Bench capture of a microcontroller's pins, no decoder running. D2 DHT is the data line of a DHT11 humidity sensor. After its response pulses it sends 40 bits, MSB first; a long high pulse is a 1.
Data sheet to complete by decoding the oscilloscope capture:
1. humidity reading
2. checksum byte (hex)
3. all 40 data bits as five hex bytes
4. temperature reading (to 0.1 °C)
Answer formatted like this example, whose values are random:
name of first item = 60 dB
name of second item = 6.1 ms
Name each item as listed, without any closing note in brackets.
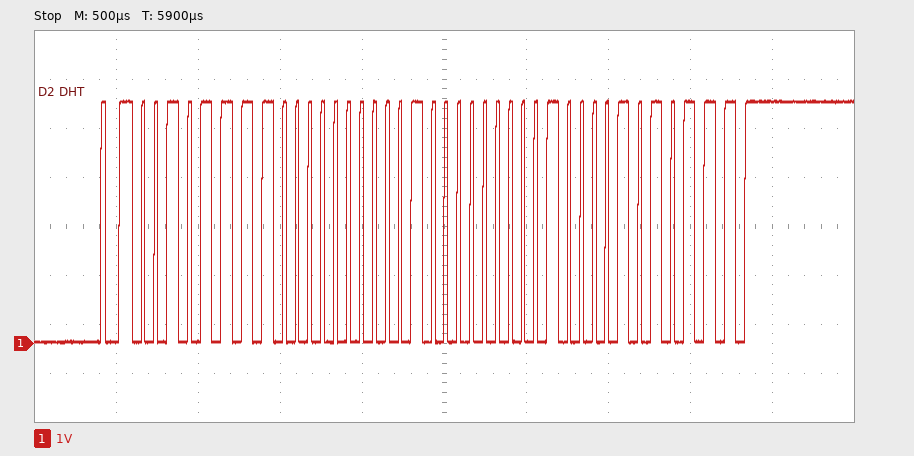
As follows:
humidity reading = 47 %
checksum byte = 0x57
all 40 data bits as five hex bytes = 2F 00 20 08 57
temperature reading = 32.8 °C
